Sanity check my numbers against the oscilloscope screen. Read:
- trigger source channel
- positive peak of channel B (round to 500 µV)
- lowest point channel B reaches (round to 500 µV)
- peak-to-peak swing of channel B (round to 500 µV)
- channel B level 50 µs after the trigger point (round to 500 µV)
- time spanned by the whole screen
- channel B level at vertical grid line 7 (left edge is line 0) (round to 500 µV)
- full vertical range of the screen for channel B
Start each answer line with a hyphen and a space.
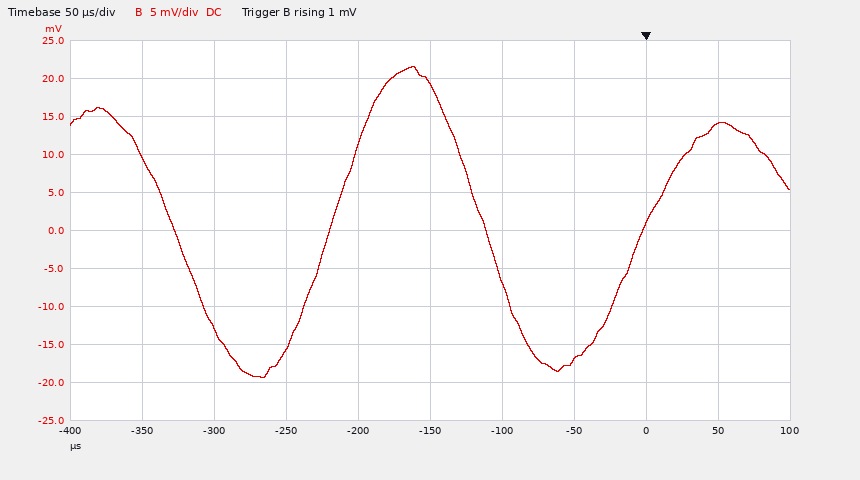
- channel B
- 21.5 mV
- -19.5 mV
- 41.0 mV
- 14.0 mV
- 500 µs
- -17.0 mV
- 50 mV
